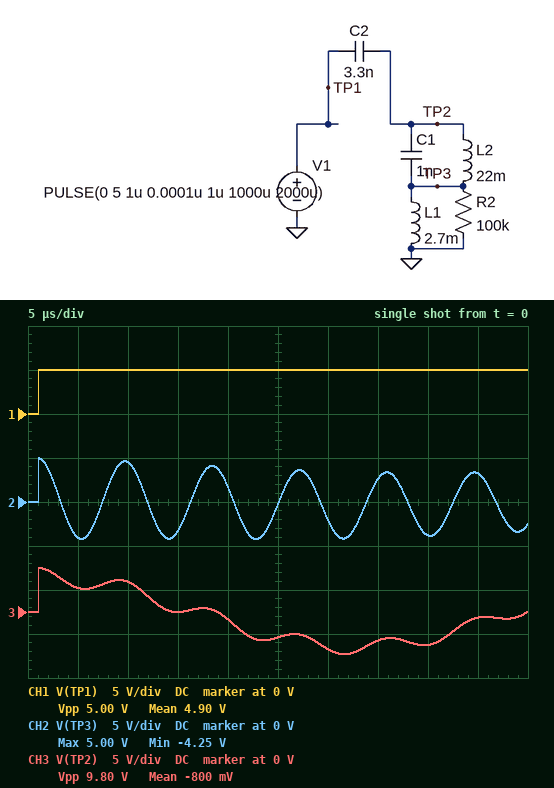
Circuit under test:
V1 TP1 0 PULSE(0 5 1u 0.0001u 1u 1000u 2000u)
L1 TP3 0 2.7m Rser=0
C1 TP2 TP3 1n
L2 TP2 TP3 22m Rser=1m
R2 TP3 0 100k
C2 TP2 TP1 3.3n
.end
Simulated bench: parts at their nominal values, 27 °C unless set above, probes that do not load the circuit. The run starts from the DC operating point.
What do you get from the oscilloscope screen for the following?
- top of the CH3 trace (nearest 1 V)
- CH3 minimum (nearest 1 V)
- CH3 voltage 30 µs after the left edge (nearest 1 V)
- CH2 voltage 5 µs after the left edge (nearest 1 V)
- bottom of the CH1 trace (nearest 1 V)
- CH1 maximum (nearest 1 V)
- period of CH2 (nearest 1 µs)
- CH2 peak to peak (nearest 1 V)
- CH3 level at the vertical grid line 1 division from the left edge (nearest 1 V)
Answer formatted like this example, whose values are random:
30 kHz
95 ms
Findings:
5 V
-5 V
-4 V
-4 V
0 V
5 V
9 µs
9 V
3 V
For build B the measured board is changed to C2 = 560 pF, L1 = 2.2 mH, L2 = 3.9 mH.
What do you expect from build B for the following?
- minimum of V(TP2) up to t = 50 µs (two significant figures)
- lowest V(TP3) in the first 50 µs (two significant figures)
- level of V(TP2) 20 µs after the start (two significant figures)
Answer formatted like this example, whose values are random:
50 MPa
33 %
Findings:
-4.7 V
-4.5 V
-1.0 V
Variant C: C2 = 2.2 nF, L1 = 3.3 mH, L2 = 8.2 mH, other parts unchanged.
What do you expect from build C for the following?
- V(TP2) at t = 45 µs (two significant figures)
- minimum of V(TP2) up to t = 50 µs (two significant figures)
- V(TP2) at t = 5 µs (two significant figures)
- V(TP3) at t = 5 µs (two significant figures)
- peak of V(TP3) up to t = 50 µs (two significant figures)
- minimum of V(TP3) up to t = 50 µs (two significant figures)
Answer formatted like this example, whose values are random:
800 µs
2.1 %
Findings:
720 mV
-4.1 V
2.0 V
-3.2 V
5.0 V
-4.3 V
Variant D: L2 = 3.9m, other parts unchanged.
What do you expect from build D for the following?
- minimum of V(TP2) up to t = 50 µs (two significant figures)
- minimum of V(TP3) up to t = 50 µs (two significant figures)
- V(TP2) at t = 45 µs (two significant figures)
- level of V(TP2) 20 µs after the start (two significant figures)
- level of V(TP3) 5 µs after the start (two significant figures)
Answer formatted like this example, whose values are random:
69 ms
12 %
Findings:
-4.5 V
-4.3 V
-3.7 V
-3.8 V
-2.1 V
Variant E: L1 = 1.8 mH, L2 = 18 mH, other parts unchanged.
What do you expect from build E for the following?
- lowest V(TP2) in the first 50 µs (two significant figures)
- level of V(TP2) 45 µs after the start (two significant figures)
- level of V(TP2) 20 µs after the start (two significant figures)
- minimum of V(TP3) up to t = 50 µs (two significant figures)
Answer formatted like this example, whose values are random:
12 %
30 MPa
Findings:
-4.6 V
1.1 V
-2.5 V
-4.3 V
